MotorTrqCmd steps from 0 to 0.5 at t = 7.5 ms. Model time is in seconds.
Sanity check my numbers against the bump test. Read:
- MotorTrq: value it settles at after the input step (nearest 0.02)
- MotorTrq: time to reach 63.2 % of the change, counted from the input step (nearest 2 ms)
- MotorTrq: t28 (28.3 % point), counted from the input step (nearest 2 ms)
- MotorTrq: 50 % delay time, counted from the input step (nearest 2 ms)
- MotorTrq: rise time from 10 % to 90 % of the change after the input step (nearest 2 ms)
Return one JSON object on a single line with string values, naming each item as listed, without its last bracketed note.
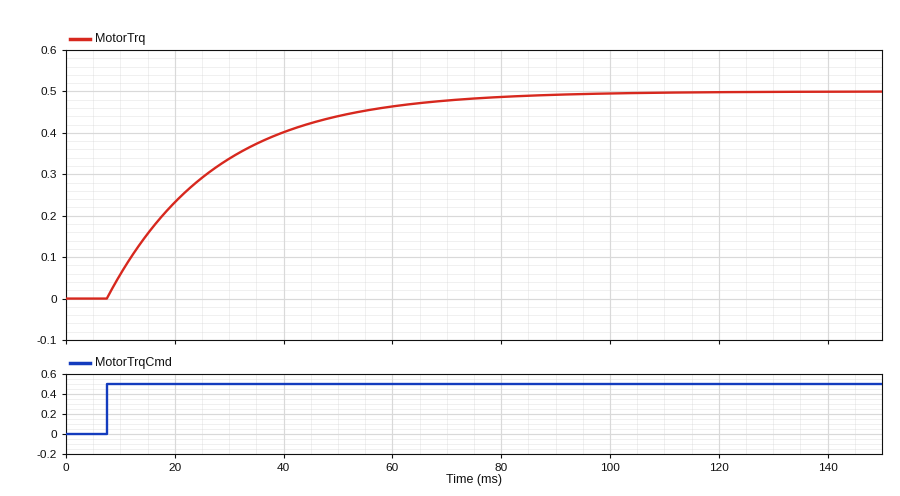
{"MotorTrq: value it settles at after the input step": "0.50", "MotorTrq: time to reach 63.2 % of the change, counted from the input step": "20 ms", "MotorTrq: t28 (28.3 % point), counted from the input step": "6 ms", "MotorTrq: 50 % delay time, counted from the input step": "14 ms", "MotorTrq: rise time from 10 % to 90 % of the change after the input step": "44 ms"}
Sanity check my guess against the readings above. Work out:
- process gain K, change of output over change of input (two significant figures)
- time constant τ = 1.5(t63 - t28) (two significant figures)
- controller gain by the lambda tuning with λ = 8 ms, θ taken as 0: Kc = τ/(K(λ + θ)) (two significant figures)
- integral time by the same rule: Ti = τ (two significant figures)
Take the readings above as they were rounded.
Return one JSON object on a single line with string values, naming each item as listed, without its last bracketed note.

{"process gain K, change of output over change of input": "1.0", "time constant τ = 1.5(t63 - t28)": "21 ms", "controller gain by the lambda tuning with λ = 8 ms, θ taken as 0: Kc = τ/(K(λ + θ))": "2.6", "integral time by the same rule: Ti = τ": "21 ms"}
